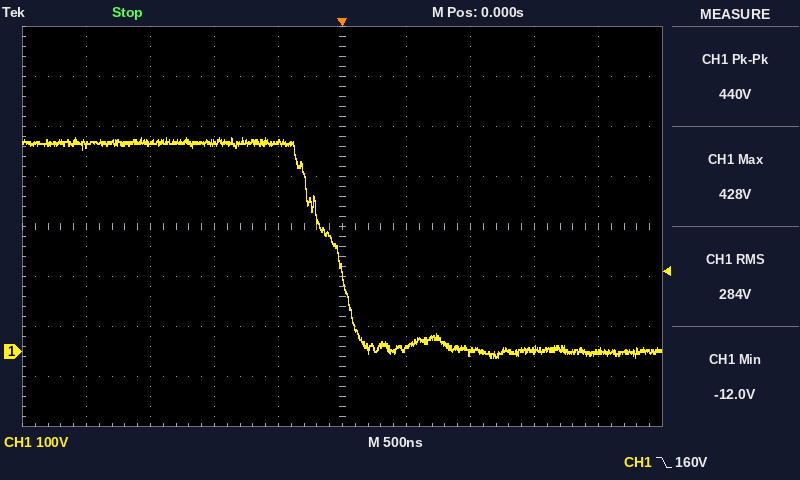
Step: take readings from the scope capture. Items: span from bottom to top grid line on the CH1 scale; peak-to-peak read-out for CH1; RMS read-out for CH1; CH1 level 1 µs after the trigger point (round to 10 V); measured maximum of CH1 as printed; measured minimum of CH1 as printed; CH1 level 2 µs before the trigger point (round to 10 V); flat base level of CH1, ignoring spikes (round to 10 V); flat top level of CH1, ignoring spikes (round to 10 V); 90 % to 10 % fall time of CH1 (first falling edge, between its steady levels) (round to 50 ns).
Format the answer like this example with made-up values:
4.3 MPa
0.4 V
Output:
800 V
440 V
284 V
0 V
428 V
-12.0 V
420 V
0 V
420 V
450 ns
